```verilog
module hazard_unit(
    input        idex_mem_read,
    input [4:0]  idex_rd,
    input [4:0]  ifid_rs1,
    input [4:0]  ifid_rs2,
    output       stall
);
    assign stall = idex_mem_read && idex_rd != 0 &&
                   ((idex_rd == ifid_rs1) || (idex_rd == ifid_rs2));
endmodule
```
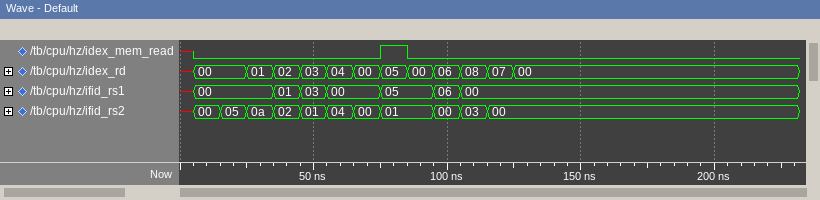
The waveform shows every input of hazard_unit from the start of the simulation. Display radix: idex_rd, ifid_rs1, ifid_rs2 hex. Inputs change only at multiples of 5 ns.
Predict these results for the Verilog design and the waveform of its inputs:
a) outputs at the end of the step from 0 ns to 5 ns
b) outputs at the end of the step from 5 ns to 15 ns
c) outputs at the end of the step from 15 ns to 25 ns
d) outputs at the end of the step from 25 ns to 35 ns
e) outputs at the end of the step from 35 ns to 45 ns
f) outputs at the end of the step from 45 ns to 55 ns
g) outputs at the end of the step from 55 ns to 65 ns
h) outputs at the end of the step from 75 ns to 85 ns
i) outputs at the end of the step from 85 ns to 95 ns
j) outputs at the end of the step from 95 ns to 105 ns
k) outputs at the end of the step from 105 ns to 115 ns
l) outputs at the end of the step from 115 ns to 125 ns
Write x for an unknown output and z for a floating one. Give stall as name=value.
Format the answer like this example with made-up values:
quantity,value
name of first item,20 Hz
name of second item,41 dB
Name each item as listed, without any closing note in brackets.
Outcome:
quantity,value
outputs at the end of the step from 0 ns to 5 ns,stall=x
outputs at the end of the step from 5 ns to 15 ns,stall=0
outputs at the end of the step from 15 ns to 25 ns,stall=0
outputs at the end of the step from 25 ns to 35 ns,stall=0
outputs at the end of the step from 35 ns to 45 ns,stall=0
outputs at the end of the step from 45 ns to 55 ns,stall=0
outputs at the end of the step from 55 ns to 65 ns,stall=0
outputs at the end of the step from 75 ns to 85 ns,stall=1
outputs at the end of the step from 85 ns to 95 ns,stall=0
outputs at the end of the step from 95 ns to 105 ns,stall=0
outputs at the end of the step from 105 ns to 115 ns,stall=0
outputs at the end of the step from 115 ns to 125 ns,stall=0
